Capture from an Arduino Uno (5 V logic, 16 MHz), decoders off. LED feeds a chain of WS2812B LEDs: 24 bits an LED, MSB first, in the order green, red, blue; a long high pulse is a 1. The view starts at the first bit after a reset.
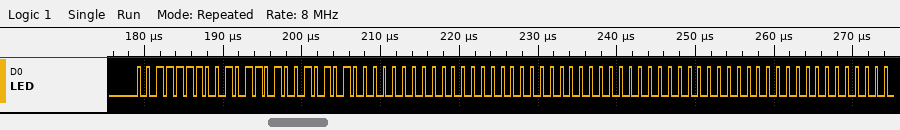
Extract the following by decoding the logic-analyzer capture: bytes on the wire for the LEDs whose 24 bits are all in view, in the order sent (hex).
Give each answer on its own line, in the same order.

3E 5A 54 00 00 00 00 00 00
